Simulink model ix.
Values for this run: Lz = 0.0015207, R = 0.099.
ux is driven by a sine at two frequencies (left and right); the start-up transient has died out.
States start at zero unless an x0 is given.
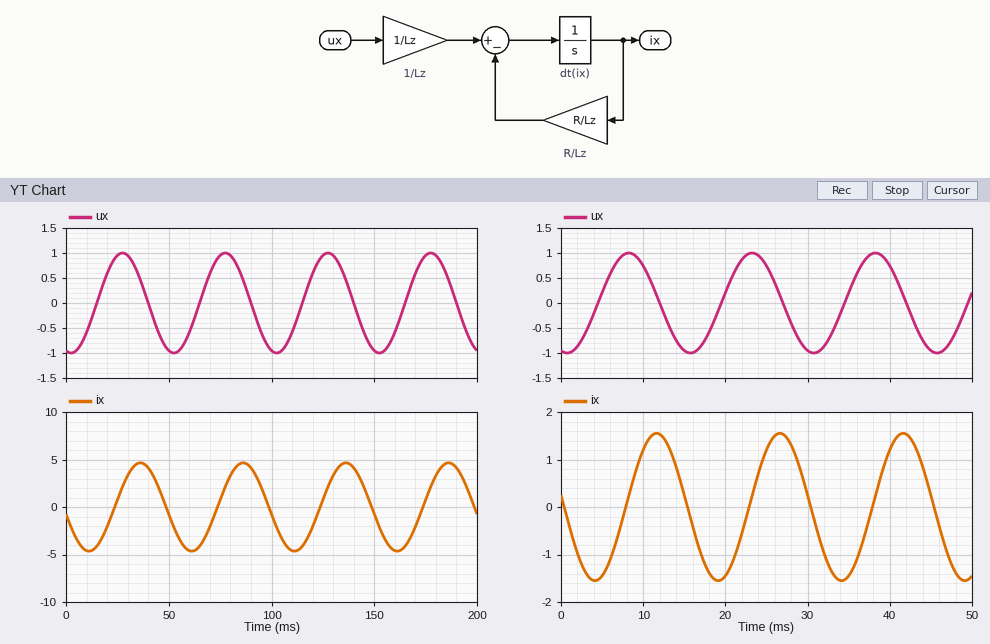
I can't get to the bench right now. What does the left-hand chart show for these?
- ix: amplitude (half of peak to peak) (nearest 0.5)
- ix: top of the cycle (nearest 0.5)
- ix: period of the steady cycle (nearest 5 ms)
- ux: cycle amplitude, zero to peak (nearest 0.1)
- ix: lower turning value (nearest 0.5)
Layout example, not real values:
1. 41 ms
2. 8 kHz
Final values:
1. 4.5
2. 4.5
3. 50 ms
4. 1.0
5. -4.5
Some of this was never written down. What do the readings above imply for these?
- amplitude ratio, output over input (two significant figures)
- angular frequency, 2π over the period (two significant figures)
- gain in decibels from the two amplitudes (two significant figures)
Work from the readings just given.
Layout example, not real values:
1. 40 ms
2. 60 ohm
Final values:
1. 4.5
2. 0.13 rad/ms
3. 13 dB
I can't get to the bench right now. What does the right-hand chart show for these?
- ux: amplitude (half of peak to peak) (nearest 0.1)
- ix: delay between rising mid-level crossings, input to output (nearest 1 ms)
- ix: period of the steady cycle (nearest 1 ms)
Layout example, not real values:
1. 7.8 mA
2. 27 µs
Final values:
1. 1.0
2. 3 ms
3. 15 ms
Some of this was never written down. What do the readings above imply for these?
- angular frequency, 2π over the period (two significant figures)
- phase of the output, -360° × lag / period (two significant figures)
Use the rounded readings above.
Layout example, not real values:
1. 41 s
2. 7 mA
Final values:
1. 0.42 rad/ms
2. -72°
